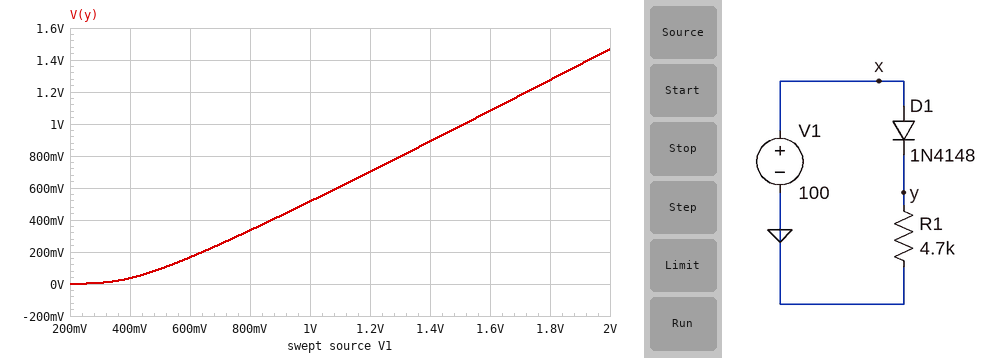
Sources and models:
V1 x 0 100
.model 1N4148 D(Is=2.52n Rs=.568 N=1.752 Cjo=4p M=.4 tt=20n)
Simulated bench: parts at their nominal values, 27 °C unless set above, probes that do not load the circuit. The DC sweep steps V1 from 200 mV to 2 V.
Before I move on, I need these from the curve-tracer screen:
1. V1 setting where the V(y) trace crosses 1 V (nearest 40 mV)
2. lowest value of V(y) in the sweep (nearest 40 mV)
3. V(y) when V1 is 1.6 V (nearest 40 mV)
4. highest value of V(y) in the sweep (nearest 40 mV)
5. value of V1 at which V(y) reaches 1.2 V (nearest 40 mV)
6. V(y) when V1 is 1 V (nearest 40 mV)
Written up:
1.52 V
0 V
1.08 V
1.48 V
1.72 V
520 mV
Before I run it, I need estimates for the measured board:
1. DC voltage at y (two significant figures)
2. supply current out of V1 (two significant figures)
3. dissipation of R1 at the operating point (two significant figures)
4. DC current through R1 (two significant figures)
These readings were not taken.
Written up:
99 V
21 mA
2.1 W
21 mA
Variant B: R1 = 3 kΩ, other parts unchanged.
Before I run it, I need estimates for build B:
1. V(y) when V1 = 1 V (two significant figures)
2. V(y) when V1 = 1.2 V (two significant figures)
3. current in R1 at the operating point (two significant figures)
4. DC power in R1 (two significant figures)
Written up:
500 mV
680 mV
33 mA
3.3 W
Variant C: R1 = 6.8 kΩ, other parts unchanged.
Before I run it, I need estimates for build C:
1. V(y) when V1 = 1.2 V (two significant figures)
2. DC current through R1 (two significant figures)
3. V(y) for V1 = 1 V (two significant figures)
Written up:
720 mV
15 mA
530 mV
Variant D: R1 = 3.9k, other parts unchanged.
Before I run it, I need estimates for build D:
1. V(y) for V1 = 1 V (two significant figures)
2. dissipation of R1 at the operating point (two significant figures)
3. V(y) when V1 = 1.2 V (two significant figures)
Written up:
510 mV
2.5 W
690 mV
